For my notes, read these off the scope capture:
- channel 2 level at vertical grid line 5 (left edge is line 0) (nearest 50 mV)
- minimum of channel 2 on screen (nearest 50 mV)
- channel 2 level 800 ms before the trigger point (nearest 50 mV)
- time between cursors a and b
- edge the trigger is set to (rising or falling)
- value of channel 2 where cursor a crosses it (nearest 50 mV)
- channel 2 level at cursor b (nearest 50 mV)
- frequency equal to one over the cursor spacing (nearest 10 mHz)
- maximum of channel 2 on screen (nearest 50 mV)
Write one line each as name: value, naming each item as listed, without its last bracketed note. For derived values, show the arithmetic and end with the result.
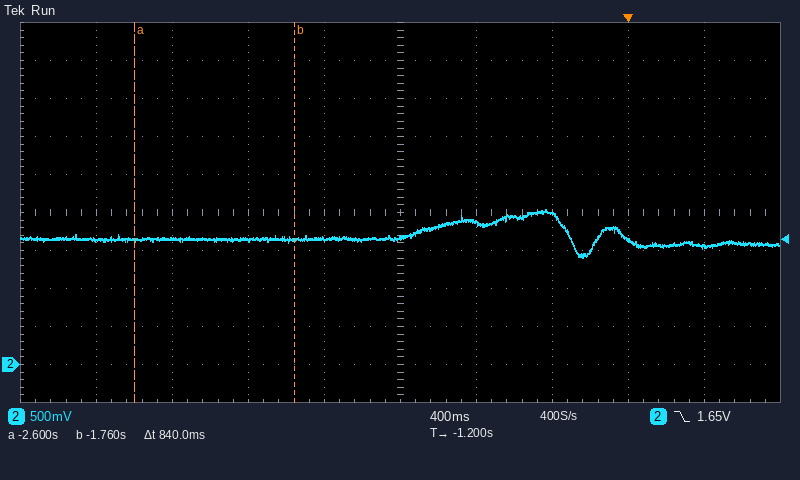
channel 2 level at vertical grid line 5 (left edge is line 0): 1.65 V
minimum of channel 2 on screen: 1.40 V
channel 2 level 800 ms before the trigger point: 1.85 V
time between cursors a and b: 840 ms
edge the trigger is set to: falling
value of channel 2 where cursor a crosses it: 1.65 V
channel 2 level at cursor b: 1.65 V
frequency equal to one over the cursor spacing: 1 / 840 ms ≈ 1.19 Hz
maximum of channel 2 on screen: 2.05 V
